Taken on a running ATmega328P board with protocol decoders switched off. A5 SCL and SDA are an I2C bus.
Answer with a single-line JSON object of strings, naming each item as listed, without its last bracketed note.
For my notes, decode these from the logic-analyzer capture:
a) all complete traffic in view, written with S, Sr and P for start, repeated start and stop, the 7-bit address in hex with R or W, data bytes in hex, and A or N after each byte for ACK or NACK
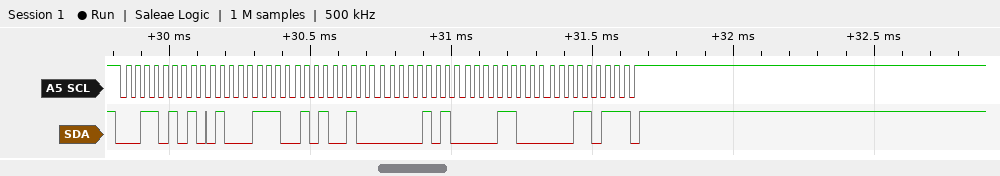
{"all complete traffic in view, written with S, Sr and P for start, repeated start and stop, the 7-bit address in hex with R or W, data bytes in hex, and A or N after each byte for ACK or NACK": "S 1AR A 47 A 52 A 05 A 0C A 1B N P"}
